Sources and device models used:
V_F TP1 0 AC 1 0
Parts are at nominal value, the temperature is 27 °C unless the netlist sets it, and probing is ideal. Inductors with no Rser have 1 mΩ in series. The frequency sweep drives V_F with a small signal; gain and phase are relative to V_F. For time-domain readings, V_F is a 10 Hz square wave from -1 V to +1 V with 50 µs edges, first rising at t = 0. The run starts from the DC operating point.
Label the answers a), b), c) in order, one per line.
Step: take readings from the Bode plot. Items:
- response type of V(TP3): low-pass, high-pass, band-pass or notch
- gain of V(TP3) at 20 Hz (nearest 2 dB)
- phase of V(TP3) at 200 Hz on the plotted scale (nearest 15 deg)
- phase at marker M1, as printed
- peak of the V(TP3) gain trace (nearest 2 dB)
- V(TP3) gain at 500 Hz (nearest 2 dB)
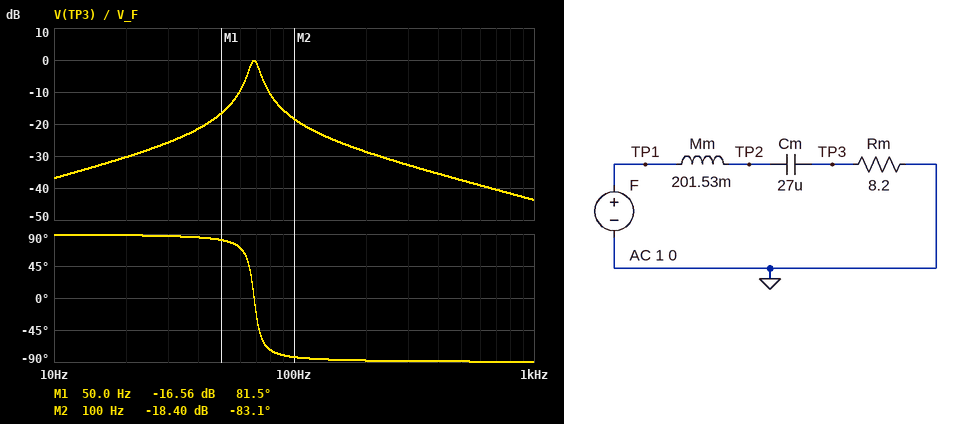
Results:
a) band-pass
b) -30 dB
c) -90 deg
d) 81.5 deg
e) 0 dB
f) -38 dB
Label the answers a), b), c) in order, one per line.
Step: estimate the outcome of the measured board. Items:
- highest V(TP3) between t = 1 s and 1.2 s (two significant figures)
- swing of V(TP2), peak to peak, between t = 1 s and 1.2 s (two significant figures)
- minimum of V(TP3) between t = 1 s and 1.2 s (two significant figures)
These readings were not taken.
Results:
a) 240 mV
b) 6.7 V
c) -240 mV
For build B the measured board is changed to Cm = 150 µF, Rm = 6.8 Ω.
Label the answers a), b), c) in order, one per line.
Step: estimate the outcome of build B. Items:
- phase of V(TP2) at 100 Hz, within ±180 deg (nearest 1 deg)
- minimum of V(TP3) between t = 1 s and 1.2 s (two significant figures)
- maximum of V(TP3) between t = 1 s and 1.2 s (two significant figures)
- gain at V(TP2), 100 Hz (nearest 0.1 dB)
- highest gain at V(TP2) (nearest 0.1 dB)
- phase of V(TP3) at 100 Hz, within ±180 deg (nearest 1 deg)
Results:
a) -144 deg
b) -510 mV
c) 510 mV
d) -19.3 dB
e) 14.8 dB
f) -87 deg
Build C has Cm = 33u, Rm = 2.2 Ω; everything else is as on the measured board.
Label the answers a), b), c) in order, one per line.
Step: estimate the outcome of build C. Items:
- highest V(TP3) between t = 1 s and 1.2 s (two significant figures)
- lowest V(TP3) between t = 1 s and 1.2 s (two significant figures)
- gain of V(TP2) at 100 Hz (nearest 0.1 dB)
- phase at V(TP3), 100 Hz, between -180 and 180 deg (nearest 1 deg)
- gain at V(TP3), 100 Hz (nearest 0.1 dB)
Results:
a) 32 mV
b) -32 mV
c) -4.2 dB
d) -88 deg
e) -31.0 dB
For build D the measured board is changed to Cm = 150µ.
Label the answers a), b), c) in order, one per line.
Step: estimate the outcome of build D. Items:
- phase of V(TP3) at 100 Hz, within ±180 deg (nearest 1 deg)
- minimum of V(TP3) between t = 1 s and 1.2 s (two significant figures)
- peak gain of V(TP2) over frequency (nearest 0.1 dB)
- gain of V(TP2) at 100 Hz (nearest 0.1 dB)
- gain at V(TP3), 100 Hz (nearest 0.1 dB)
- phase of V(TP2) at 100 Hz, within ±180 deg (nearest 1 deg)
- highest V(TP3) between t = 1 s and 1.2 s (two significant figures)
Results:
a) -86 deg
b) -550 mV
c) 13.3 dB
d) -18.8 dB
e) -23.0 dB
f) -138 deg
g) 550 mV
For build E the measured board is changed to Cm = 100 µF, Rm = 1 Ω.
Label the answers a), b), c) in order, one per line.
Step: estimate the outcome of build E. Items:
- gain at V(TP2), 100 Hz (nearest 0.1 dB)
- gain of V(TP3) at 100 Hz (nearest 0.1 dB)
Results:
a) -16.8 dB
b) -40.9 dB
